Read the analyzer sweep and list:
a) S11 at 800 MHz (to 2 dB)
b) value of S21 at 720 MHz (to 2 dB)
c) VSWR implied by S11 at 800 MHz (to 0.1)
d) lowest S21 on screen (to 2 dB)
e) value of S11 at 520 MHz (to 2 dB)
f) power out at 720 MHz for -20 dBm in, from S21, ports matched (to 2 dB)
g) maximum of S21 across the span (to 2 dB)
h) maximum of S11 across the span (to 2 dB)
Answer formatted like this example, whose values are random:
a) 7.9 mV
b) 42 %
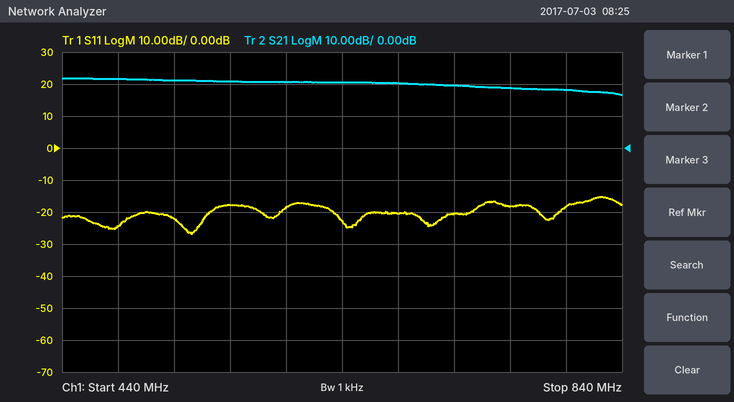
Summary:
a) -18 dB
b) 20 dB
c) 1.3
d) 16 dB
e) -22 dB
f) 0 dBm
g) 22 dB
h) -16 dB
